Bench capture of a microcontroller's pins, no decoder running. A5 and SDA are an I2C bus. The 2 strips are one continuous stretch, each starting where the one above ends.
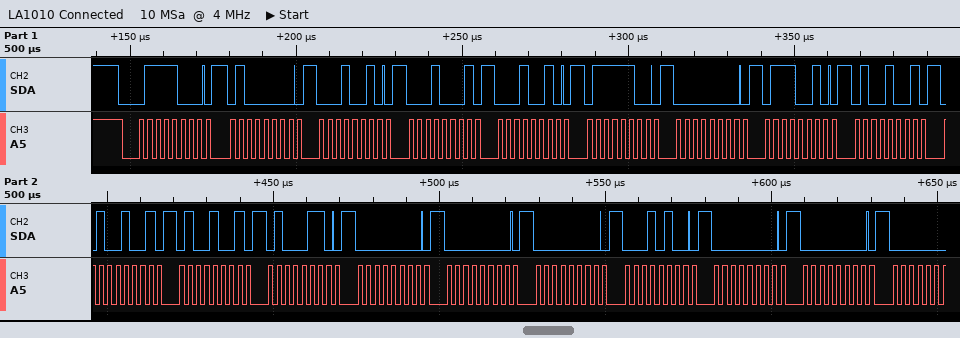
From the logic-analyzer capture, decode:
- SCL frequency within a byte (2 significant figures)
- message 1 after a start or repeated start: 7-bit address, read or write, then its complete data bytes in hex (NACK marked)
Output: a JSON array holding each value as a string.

["400 kHz", "0x3C write: 40 12 11 12 7C 00 72 49 49 49 46 00 00 00 14 00 00"]
